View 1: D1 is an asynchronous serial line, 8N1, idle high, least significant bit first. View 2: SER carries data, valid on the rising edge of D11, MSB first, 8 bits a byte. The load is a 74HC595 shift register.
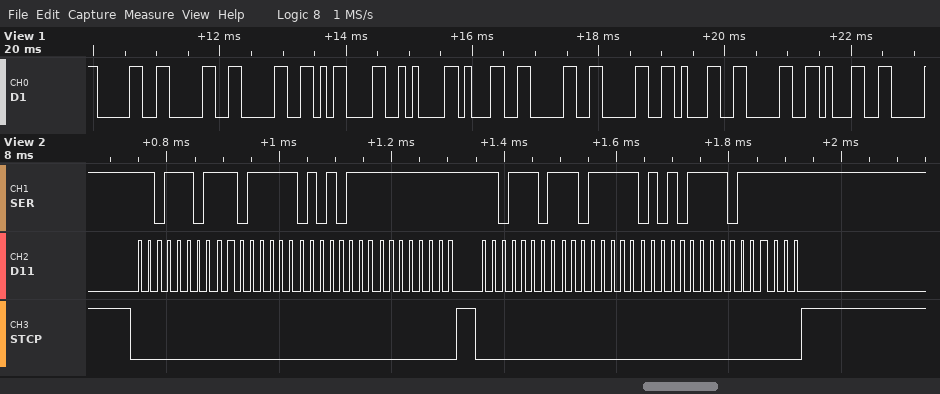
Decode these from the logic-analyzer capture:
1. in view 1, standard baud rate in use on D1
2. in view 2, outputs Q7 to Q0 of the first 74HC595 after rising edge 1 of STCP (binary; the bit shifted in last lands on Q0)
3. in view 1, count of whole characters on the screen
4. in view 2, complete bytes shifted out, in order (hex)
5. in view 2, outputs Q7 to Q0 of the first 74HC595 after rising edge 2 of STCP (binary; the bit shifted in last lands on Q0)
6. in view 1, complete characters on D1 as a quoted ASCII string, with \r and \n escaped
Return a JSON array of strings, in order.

["9600 baud", "11111111", "11", "0xDD 0xDF 0x57 0xFF 0xDD 0xDF 0x57 0xBF", "10111111", "\"000\\r\\n100101\""]
